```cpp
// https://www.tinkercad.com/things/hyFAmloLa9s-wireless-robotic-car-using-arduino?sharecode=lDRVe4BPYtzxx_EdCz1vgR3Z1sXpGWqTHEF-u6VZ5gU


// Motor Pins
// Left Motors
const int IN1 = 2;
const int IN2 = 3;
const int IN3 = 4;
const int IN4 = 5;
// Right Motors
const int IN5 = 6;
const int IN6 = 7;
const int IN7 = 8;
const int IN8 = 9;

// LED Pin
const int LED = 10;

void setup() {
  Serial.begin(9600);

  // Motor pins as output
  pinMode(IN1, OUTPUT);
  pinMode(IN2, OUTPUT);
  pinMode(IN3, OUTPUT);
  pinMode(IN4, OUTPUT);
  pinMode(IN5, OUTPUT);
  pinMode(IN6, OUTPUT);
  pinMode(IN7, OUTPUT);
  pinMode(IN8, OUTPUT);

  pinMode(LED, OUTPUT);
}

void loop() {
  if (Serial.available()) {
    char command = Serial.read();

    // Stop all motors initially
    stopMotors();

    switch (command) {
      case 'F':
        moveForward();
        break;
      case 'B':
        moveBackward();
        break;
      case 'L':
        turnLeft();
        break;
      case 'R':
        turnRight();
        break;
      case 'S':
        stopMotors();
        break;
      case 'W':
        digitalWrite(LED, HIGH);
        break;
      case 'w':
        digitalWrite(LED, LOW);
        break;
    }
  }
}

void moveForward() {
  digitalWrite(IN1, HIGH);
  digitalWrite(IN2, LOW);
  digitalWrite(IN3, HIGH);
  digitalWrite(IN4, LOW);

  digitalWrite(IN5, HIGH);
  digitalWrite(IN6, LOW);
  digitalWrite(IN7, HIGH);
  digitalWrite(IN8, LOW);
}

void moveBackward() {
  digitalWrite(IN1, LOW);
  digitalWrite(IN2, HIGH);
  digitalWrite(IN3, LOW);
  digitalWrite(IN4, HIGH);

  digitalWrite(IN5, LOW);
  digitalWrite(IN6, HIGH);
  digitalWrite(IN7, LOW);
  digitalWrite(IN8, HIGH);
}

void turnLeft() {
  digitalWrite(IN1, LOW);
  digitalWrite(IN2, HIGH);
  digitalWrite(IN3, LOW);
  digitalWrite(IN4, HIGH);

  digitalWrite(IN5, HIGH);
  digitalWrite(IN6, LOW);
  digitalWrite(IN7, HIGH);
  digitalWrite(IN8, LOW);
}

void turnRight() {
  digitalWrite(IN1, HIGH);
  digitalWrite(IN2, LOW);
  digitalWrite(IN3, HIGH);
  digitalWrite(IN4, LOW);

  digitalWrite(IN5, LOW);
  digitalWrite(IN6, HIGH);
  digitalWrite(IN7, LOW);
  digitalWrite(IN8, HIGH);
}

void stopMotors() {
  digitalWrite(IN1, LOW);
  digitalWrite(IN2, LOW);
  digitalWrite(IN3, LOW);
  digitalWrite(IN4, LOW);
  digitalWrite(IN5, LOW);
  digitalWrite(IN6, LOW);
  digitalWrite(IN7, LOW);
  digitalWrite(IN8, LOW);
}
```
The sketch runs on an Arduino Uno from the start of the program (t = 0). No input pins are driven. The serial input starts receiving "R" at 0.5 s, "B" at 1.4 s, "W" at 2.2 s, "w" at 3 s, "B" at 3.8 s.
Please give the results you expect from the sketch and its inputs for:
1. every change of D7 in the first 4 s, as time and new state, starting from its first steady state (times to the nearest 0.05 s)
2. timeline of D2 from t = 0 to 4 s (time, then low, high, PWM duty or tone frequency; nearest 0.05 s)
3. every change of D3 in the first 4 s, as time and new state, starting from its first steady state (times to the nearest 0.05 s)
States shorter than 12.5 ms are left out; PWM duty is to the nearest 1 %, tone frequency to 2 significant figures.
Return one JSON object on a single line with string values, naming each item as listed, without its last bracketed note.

{"every change of D7 in the first 4 s, as time and new state, starting from its first steady state": "0 s low; 0.5 s high; 2.2 s low; 3.8 s high", "timeline of D2 from t = 0 to 4 s": "0 s low; 0.5 s high; 1.4 s low", "every change of D3 in the first 4 s, as time and new state, starting from its first steady state": "0 s low; 1.4 s high; 2.2 s low; 3.8 s high"}
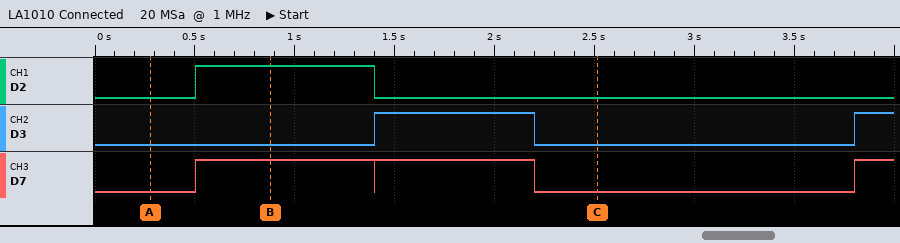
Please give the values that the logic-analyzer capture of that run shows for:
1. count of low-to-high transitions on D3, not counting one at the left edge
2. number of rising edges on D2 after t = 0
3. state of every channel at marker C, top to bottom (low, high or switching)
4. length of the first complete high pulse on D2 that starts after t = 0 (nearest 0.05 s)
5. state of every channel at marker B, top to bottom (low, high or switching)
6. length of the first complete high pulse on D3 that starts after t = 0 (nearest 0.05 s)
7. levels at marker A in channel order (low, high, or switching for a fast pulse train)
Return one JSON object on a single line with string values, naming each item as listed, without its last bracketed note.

{"count of low-to-high transitions on D3, not counting one at the left edge": "2", "number of rising edges on D2 after t = 0": "1", "state of every channel at marker C, top to bottom": "D2 low, D3 low, D7 low", "length of the first complete high pulse on D2 that starts after t = 0": "0.90 s", "state of every channel at marker B, top to bottom": "D2 high, D3 low, D7 high", "length of the first complete high pulse on D3 that starts after t = 0": "0.80 s", "levels at marker A in channel order": "D2 low, D3 low, D7 low"}
